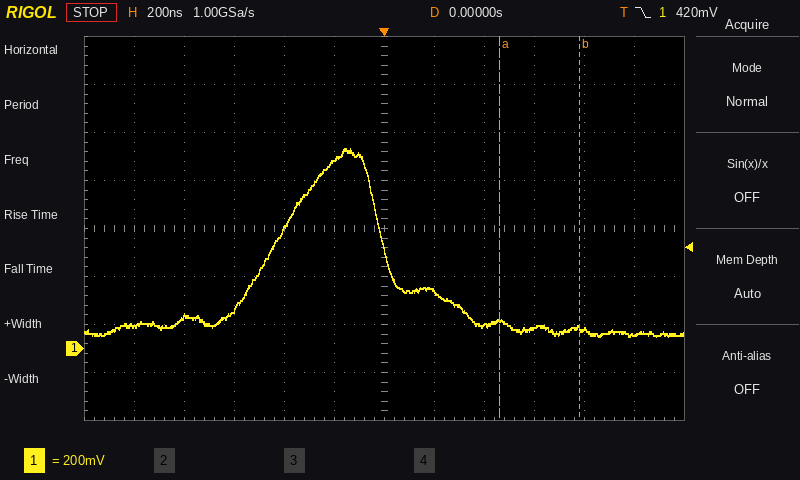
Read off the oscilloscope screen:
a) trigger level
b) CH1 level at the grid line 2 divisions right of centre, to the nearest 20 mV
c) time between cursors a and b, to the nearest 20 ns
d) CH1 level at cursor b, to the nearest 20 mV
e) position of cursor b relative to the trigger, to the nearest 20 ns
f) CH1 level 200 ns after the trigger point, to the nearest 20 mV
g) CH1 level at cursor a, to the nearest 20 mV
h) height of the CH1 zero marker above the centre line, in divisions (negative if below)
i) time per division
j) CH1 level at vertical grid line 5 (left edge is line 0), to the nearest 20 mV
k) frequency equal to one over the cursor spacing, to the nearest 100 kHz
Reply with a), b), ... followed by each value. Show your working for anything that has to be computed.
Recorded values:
a) 420 mV
b) 100 mV
c) 320 ns
d) 80 mV
e) +780 ns
f) 240 mV
g) 120 mV
h) -2.5 div
i) 200 ns
j) 780 mV
k) 1 / 320 ns ≈ 3.1 MHz
